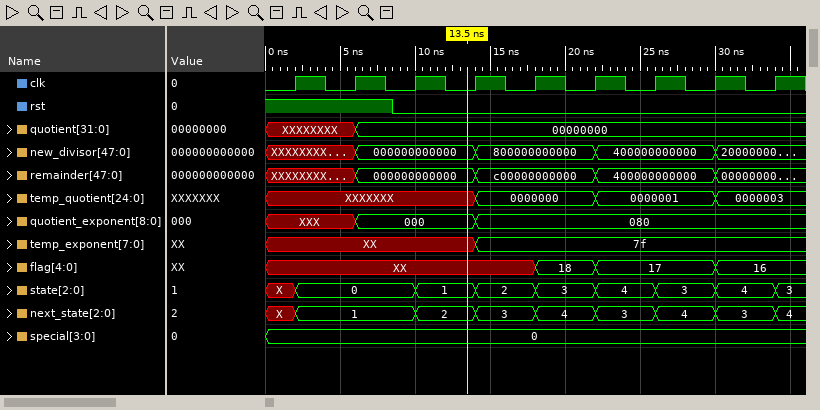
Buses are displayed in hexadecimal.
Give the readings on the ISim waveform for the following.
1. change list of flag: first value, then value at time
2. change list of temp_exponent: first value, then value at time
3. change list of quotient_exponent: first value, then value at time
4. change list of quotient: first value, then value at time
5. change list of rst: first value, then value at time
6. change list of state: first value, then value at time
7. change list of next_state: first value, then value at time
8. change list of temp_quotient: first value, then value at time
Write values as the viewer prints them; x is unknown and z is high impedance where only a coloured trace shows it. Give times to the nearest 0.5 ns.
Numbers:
XX, 18 at 18 ns, 17 at 22 ns, 16 at 30 ns
XX, 7f at 14 ns
XXX, 000 at 6 ns, 080 at 14 ns
XXXXXXXX, 00000000 at 6 ns
1, 0 at 8.5 ns
X, 0 at 2 ns, 1 at 10 ns, 2 at 14 ns, 3 at 18 ns, 4 at 22 ns, 3 at 26 ns, 4 at 30 ns, 3 at 34 ns
X, 1 at 2 ns, 2 at 10 ns, 3 at 14 ns, 4 at 18 ns, 3 at 22 ns, 4 at 26 ns, 3 at 30 ns, 4 at 34 ns
XXXXXXX, 0000000 at 14 ns, 0000001 at 22 ns, 0000003 at 30 ns
